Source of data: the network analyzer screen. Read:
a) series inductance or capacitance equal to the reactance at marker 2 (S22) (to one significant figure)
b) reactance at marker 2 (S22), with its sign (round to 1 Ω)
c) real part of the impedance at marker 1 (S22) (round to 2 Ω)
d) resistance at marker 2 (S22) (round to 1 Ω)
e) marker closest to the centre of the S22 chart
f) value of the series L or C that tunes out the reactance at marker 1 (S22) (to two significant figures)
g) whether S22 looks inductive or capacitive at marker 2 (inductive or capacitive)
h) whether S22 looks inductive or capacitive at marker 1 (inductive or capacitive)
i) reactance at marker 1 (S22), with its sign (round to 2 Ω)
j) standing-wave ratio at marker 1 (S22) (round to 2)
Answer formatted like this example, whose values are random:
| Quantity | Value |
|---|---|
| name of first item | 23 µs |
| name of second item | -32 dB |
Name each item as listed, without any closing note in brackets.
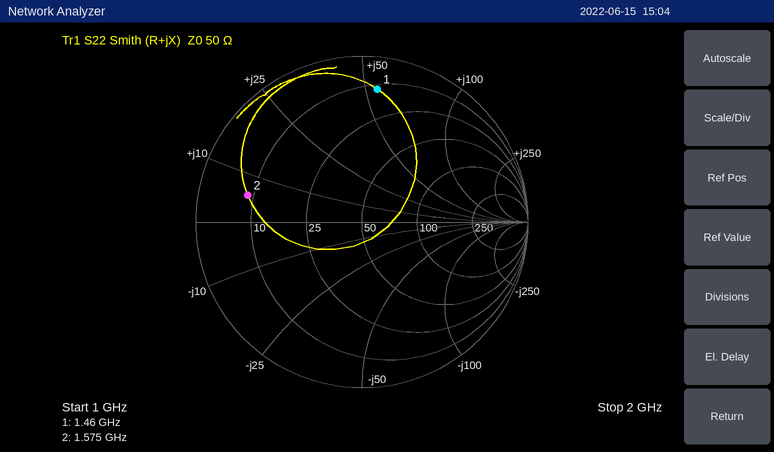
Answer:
| Quantity | Value |
|---|---|
| series inductance or capacitance equal to the reactance at marker 2 (S22) | 600 pH |
| reactance at marker 2 (S22), with its sign | +6 Ω |
| real part of the impedance at marker 1 (S22) | 12 Ω |
| resistance at marker 2 (S22) | 9 Ω |
| marker closest to the centre of the S22 chart | marker 2 |
| value of the series L or C that tunes out the reactance at marker 1 (S22) | 2.0 pF |
| whether S22 looks inductive or capacitive at marker 2 | inductive |
| whether S22 looks inductive or capacitive at marker 1 | inductive |
| reactance at marker 1 (S22), with its sign | +54 Ω |
| standing-wave ratio at marker 1 (S22) | 10 |
